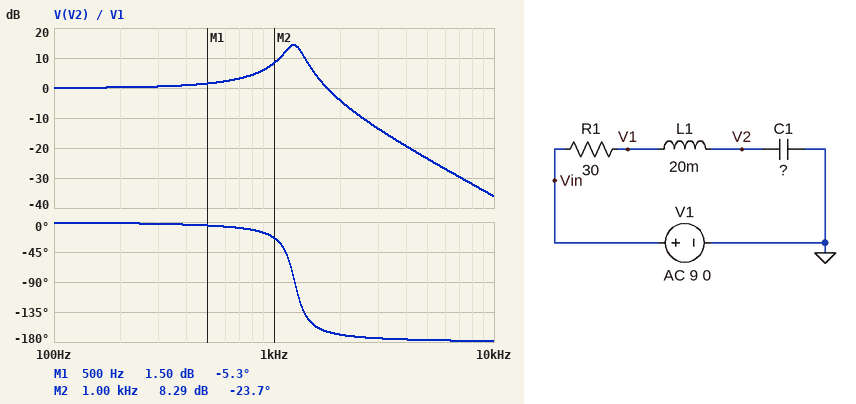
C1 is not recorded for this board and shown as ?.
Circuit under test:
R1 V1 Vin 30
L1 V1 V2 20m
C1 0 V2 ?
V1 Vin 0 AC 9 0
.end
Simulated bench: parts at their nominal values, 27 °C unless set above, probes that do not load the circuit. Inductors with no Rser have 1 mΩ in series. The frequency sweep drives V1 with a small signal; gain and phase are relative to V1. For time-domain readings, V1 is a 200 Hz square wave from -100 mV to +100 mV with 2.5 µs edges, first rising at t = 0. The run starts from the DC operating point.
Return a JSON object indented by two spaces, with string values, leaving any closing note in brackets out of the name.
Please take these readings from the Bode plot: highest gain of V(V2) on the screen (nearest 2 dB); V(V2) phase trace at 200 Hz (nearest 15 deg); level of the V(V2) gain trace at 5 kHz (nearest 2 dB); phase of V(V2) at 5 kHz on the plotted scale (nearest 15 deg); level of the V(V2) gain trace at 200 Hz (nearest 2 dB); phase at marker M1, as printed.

{
  "highest gain of V(V2) on the screen": "14 dB",
  "V(V2) phase trace at 200 Hz": "0 deg",
  "level of the V(V2) gain trace at 5 kHz": "-24 dB",
  "phase of V(V2) at 5 kHz on the plotted scale": "-180 deg",
  "level of the V(V2) gain trace at 200 Hz": "0 dB",
  "phase at marker M1, as printed": "-5.3 deg"
}
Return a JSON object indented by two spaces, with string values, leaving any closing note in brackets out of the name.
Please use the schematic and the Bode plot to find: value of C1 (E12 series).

{
  "value of C1": "820 nF"
}
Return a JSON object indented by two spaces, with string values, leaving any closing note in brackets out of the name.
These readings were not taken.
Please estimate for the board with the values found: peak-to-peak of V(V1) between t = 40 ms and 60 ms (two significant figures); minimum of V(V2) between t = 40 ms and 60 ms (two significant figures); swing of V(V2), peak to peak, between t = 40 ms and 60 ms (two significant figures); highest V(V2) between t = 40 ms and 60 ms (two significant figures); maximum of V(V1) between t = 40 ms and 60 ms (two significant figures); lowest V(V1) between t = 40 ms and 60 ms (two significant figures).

{
  "peak-to-peak of V(V1) between t = 40 ms and 60 ms": "240 mV",
  "minimum of V(V2) between t = 40 ms and 60 ms": "-230 mV",
  "swing of V(V2), peak to peak, between t = 40 ms and 60 ms": "460 mV",
  "highest V(V2) between t = 40 ms and 60 ms": "230 mV",
  "maximum of V(V1) between t = 40 ms and 60 ms": "120 mV",
  "lowest V(V1) between t = 40 ms and 60 ms": "-120 mV"
}
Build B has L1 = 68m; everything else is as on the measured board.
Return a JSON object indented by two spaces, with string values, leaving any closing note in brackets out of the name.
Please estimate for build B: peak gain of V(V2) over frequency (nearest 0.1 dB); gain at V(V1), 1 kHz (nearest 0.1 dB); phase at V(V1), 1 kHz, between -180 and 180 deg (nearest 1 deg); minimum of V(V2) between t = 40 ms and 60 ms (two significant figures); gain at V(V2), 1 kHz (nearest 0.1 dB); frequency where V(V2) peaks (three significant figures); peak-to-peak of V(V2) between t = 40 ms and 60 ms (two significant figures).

{
  "peak gain of V(V2) over frequency": "19.7 dB",
  "gain at V(V1), 1 kHz": "-0.1 dB",
  "phase at V(V1), 1 kHz, between -180 and 180 deg": "7 deg",
  "minimum of V(V2) between t = 40 ms and 60 ms": "-290 mV",
  "gain at V(V2), 1 kHz": "-1.7 dB",
  "frequency where V(V2) peaks": "672 Hz",
  "peak-to-peak of V(V2) between t = 40 ms and 60 ms": "580 mV"
}
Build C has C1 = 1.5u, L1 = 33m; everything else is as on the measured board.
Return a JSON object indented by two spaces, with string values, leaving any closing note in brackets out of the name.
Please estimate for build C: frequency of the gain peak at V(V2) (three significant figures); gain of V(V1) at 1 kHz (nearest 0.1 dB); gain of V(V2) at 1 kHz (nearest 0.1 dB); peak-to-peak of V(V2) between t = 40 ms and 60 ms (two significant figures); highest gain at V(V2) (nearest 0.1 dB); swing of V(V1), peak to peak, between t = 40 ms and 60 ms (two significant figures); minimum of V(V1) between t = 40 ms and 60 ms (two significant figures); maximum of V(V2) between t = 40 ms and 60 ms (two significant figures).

{
  "frequency of the gain peak at V(V2)": "708 Hz",
  "gain of V(V1) at 1 kHz": "-0.4 dB",
  "gain of V(V2) at 1 kHz": "0 dB",
  "peak-to-peak of V(V2) between t = 40 ms and 60 ms": "470 mV",
  "highest gain at V(V2)": "13.9 dB",
  "swing of V(V1), peak to peak, between t = 40 ms and 60 ms": "250 mV",
  "minimum of V(V1) between t = 40 ms and 60 ms": "-120 mV",
  "maximum of V(V2) between t = 40 ms and 60 ms": "240 mV"
}
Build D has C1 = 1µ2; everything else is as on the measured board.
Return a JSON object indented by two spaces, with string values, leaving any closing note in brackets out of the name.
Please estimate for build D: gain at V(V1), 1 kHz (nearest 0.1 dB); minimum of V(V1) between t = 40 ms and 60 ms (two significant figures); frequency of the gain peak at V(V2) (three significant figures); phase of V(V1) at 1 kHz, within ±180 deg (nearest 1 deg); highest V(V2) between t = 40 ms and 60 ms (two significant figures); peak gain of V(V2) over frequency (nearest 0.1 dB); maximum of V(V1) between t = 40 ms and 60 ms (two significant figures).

{
  "gain at V(V1), 1 kHz": "-12.9 dB",
  "minimum of V(V1) between t = 40 ms and 60 ms": "-130 mV",
  "frequency of the gain peak at V(V2)": "1.01 kHz",
  "phase of V(V1) at 1 kHz, within ±180 deg": "-77 deg",
  "highest V(V2) between t = 40 ms and 60 ms": "260 mV",
  "peak gain of V(V2) over frequency": "12.7 dB",
  "maximum of V(V1) between t = 40 ms and 60 ms": "130 mV"
}
